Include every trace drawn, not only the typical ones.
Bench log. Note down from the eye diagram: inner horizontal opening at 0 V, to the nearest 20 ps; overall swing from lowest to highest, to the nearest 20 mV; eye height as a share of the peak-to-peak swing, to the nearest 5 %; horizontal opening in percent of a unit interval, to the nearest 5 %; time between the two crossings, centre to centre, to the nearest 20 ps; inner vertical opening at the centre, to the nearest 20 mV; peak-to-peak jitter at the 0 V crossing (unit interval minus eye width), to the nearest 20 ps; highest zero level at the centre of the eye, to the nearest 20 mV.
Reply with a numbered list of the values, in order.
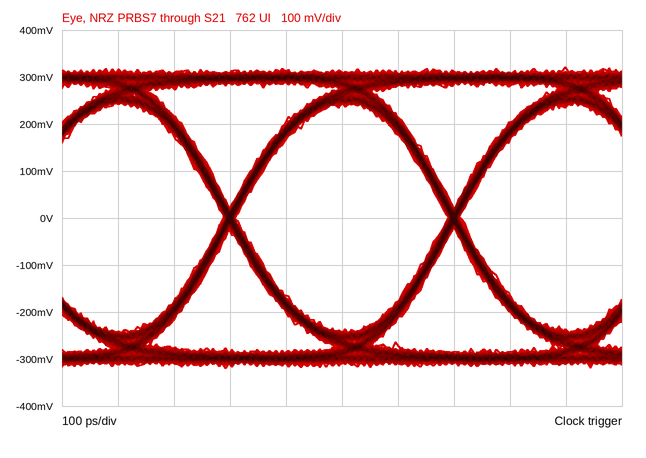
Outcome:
1. 380 ps
2. 640 mV
3. 75 %
4. 95 %
5. 400 ps
6. 480 mV
7. 20 ps
8. -240 mV
